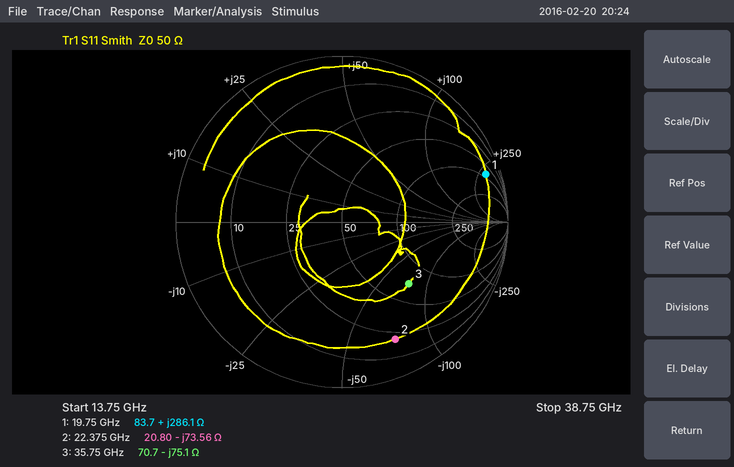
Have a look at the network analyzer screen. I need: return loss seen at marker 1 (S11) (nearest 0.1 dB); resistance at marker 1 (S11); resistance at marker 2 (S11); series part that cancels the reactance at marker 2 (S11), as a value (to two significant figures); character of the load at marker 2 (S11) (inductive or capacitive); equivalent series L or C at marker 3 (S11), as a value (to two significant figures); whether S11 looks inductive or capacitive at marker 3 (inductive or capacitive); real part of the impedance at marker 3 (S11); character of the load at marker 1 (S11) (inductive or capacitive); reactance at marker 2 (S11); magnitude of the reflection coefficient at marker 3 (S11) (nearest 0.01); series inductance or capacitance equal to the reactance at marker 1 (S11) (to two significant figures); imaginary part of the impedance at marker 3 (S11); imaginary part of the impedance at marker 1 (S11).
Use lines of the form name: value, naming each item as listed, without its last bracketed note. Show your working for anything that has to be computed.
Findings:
return loss seen at marker 1 (S11): 0.8 dB
resistance at marker 1: 83.7 Ω
resistance at marker 2: 20.80 Ω
series part that cancels the reactance at marker 2 (S11), as a value: L = 73.56 Ω/(2π × 22.375 GHz) ≈ 523 pH, so 520 pH to two significant figures
character of the load at marker 2 (S11): capacitive
equivalent series L or C at marker 3 (S11), as a value: C = 1/(2π × 35.75 GHz × 75.1 Ω) ≈ 59 fF
whether S11 looks inductive or capacitive at marker 3: capacitive
real part of the impedance at marker 3: 70.7 Ω
character of the load at marker 1 (S11): inductive
reactance at marker 2: -73.56 Ω
magnitude of the reflection coefficient at marker 3 (S11): 0.55
series inductance or capacitance equal to the reactance at marker 1 (S11): L = 286.1 Ω/(2π × 19.75 GHz) ≈ 2.3 nH
imaginary part of the impedance at marker 3: -75.1 Ω
imaginary part of the impedance at marker 1: +286.1 Ω
